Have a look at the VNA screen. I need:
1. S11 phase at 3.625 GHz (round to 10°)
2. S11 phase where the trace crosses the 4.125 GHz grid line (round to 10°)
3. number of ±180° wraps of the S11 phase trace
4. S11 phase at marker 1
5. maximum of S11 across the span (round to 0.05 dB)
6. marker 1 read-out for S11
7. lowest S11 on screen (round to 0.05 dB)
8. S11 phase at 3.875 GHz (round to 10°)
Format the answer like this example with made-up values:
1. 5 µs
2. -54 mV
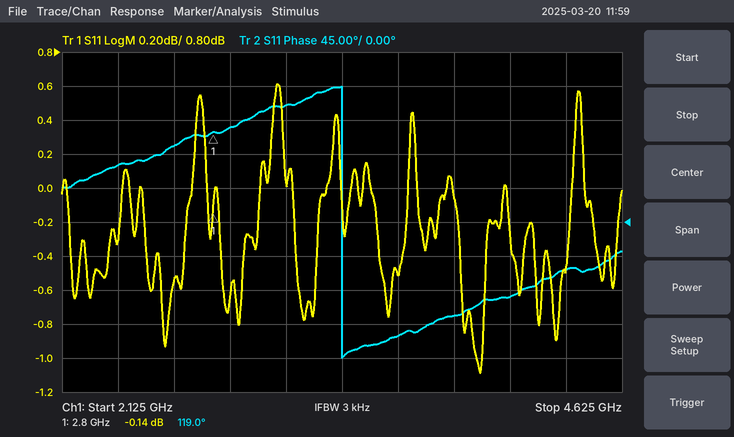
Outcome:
1. -150°
2. -100°
3. 1
4. 119.0°
5. 0.60 dB
6. -0.14 dB
7. -1.10 dB
8. -120°
